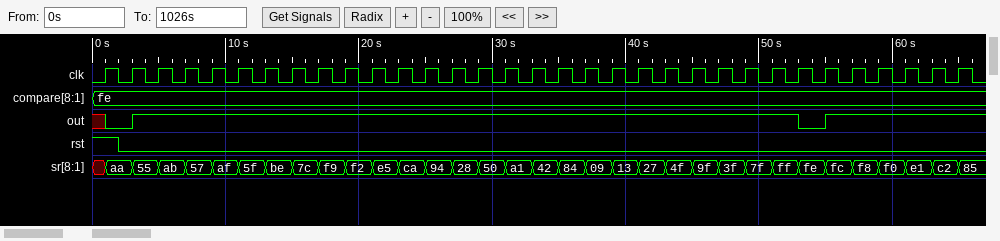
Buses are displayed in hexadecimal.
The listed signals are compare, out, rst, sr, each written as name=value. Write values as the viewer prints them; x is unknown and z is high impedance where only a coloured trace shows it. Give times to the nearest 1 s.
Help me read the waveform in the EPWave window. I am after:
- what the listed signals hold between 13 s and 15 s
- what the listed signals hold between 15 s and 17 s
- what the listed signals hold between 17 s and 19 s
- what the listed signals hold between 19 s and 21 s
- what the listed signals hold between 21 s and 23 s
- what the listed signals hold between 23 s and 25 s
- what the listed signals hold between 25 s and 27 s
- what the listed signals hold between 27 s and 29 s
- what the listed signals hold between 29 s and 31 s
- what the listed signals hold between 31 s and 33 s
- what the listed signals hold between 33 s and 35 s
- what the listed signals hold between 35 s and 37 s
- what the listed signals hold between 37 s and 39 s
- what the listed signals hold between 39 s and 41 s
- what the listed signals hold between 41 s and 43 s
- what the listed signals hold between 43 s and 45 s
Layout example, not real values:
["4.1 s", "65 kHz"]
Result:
["compare=fe, out=1, rst=0, sr=be", "compare=fe, out=1, rst=0, sr=7c", "compare=fe, out=1, rst=0, sr=f9", "compare=fe, out=1, rst=0, sr=f2", "compare=fe, out=1, rst=0, sr=e5", "compare=fe, out=1, rst=0, sr=ca", "compare=fe, out=1, rst=0, sr=94", "compare=fe, out=1, rst=0, sr=28", "compare=fe, out=1, rst=0, sr=50", "compare=fe, out=1, rst=0, sr=a1", "compare=fe, out=1, rst=0, sr=42", "compare=fe, out=1, rst=0, sr=84", "compare=fe, out=1, rst=0, sr=09", "compare=fe, out=1, rst=0, sr=13", "compare=fe, out=1, rst=0, sr=27", "compare=fe, out=1, rst=0, sr=4f"]
